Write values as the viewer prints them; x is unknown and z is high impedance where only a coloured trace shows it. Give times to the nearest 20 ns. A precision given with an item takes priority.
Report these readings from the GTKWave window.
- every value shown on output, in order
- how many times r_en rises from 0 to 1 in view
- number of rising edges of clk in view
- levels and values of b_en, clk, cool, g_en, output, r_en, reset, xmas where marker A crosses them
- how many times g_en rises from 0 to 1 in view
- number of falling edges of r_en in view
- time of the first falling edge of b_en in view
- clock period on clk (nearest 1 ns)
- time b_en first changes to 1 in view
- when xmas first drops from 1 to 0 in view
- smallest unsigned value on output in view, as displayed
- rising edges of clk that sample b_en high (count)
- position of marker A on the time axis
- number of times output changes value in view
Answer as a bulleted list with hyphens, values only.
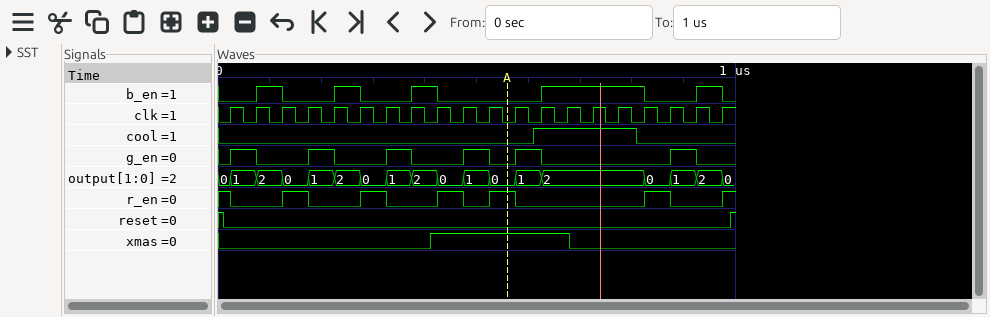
- 0, 1, 2, 0, 1, 2, 0, 1, 2, 0, 1, 0, 1, 2, 0, 1, 2, 0
- 6
- 20
- b_en=0, clk=0, cool=0, g_en=0, output=0, r_en=1, reset=0, xmas=1
- 6
- 6
- 120 ns
- 50 ns
- 80 ns
- 680 ns
- 0
- 8
- 560 ns
- 17
